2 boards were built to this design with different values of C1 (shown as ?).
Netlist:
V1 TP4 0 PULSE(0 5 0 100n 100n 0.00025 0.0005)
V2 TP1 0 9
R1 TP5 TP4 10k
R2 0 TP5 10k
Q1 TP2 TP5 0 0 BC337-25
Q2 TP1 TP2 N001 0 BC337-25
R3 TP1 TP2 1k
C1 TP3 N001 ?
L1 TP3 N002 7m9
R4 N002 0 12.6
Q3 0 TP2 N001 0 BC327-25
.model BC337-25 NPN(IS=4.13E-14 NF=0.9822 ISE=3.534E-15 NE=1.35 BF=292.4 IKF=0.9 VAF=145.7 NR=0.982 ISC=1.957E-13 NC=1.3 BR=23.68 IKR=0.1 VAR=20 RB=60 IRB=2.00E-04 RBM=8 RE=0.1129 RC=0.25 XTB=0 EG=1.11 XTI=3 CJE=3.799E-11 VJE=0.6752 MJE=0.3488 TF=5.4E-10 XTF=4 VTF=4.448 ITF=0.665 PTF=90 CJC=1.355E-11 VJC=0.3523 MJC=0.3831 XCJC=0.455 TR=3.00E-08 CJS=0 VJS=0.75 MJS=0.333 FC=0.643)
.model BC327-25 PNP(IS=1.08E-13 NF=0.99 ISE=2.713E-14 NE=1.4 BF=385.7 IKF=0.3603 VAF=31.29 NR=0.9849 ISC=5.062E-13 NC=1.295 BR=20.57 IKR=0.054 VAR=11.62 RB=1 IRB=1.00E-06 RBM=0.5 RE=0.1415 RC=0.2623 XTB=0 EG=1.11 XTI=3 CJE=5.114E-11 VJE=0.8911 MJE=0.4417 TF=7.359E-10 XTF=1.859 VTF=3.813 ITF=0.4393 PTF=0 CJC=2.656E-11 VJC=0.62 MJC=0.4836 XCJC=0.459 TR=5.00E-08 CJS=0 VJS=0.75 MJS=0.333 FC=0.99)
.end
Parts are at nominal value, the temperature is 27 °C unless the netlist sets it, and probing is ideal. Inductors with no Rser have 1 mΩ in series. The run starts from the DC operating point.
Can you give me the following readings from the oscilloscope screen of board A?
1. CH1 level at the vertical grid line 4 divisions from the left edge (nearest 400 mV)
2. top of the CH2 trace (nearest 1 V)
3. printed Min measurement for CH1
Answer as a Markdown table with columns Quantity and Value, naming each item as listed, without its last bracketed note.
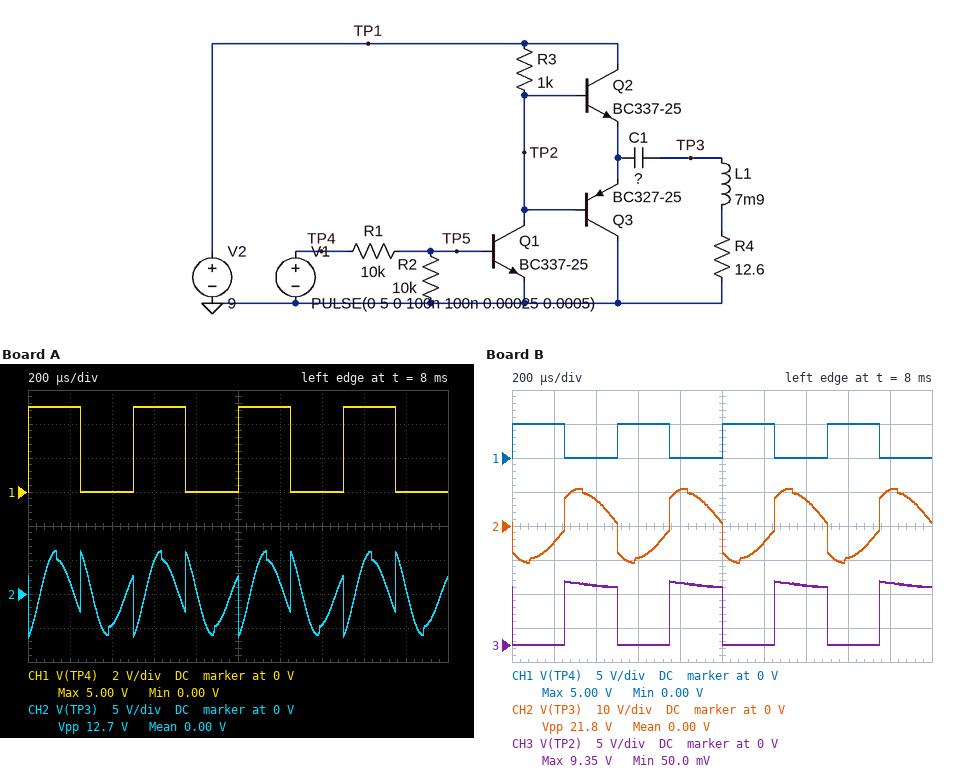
| Quantity | Value |
|---|---|
| CH1 level at the vertical grid line 4 divisions from the left edge | 0 V |
| top of the CH2 trace | 6 V |
| printed Min measurement for CH1 | 0.00 V |
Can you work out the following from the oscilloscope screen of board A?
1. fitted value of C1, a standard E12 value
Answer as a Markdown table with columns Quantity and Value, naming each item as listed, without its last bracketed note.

| Quantity | Value |
|---|---|
| fitted value of C1, a standard E12 value | 330 nF |
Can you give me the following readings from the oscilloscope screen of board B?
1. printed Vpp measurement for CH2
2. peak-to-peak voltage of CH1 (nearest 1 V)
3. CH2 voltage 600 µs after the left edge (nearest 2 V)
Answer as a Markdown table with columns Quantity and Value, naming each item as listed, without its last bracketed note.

| Quantity | Value |
|---|---|
| printed Vpp measurement for CH2 | 21.8 V |
| peak-to-peak voltage of CH1 | 5 V |
| CH2 voltage 600 µs after the left edge | -10 V |
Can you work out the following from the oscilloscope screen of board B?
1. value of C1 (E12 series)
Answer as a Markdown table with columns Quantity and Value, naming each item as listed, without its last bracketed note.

| Quantity | Value |
|---|---|
| value of C1 | 1.5 µF |
